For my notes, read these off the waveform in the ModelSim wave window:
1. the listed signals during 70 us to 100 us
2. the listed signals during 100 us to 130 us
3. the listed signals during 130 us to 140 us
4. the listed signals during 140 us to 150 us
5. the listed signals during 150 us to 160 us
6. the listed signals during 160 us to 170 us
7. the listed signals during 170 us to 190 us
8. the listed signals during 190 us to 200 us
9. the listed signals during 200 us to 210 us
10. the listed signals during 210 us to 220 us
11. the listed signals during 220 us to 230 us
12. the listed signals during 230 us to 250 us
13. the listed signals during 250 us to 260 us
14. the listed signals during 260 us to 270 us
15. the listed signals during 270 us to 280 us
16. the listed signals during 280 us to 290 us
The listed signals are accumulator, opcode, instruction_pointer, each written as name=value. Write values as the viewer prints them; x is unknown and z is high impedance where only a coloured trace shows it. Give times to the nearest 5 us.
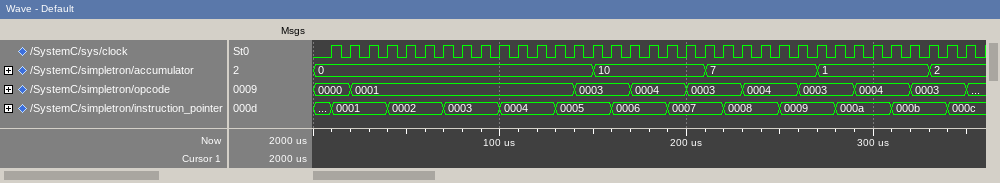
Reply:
accumulator=0, opcode=0001, instruction_pointer=0003
accumulator=0, opcode=0001, instruction_pointer=0004
accumulator=0, opcode=0001, instruction_pointer=0005
accumulator=0, opcode=0003, instruction_pointer=0005
accumulator=10, opcode=0003, instruction_pointer=0005
accumulator=10, opcode=0003, instruction_pointer=0006
accumulator=10, opcode=0004, instruction_pointer=0006
accumulator=10, opcode=0004, instruction_pointer=0007
accumulator=10, opcode=0003, instruction_pointer=0007
accumulator=7, opcode=0003, instruction_pointer=0007
accumulator=7, opcode=0003, instruction_pointer=0008
accumulator=7, opcode=0004, instruction_pointer=0008
accumulator=7, opcode=0004, instruction_pointer=0009
accumulator=7, opcode=0003, instruction_pointer=0009
accumulator=1, opcode=0003, instruction_pointer=0009
accumulator=1, opcode=0003, instruction_pointer=000a
